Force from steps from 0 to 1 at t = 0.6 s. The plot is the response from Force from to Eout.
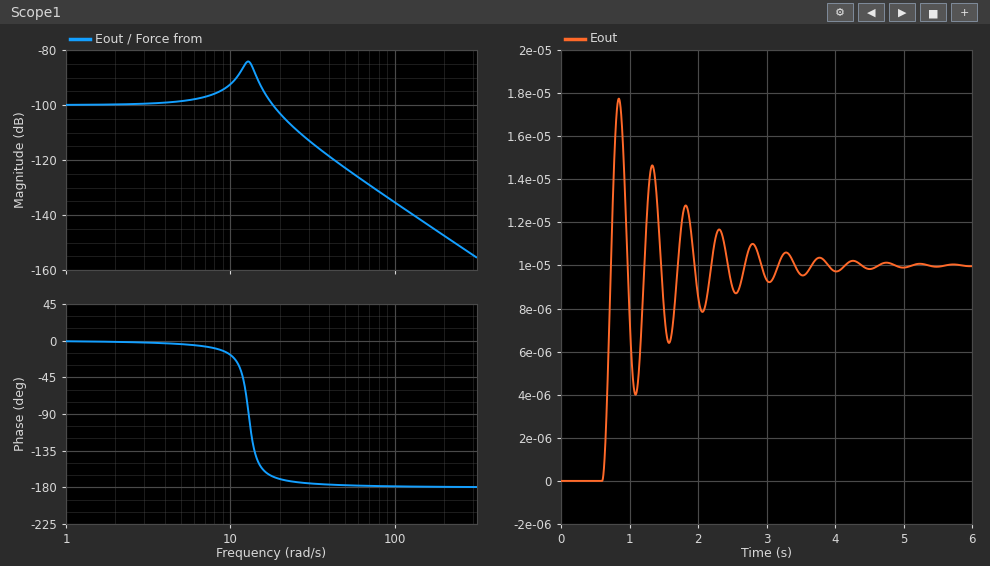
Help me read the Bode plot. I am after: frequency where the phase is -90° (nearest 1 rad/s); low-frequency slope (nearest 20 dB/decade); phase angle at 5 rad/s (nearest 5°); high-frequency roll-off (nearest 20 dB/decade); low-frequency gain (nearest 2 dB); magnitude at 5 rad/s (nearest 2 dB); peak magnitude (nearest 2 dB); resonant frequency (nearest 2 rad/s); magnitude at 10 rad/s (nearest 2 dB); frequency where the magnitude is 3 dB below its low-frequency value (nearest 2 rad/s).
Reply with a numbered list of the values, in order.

1. 13 rad/s
2. 0 dB/decade
3. -5°
4. -40 dB/decade
5. -100 dB
6. -98 dB
7. -84 dB
8. 12 rad/s
9. -92 dB
10. 20 rad/s
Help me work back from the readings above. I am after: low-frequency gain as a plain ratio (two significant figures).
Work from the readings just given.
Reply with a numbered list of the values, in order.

1. 0.000010
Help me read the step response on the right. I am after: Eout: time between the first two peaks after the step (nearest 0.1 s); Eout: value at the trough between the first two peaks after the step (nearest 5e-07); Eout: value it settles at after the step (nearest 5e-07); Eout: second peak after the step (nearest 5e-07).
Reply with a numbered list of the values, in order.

1. 0.5 s
2. 0.0000040
3. 0.0000100
4. 0.0000145
